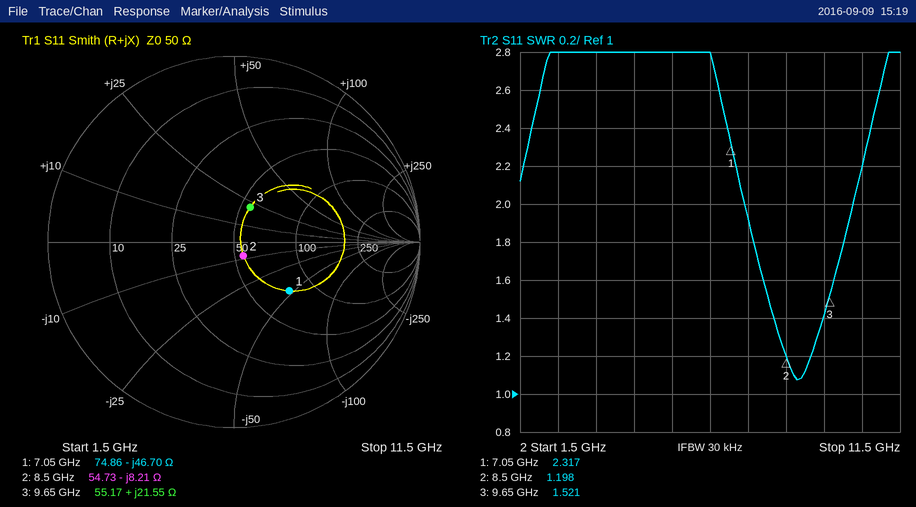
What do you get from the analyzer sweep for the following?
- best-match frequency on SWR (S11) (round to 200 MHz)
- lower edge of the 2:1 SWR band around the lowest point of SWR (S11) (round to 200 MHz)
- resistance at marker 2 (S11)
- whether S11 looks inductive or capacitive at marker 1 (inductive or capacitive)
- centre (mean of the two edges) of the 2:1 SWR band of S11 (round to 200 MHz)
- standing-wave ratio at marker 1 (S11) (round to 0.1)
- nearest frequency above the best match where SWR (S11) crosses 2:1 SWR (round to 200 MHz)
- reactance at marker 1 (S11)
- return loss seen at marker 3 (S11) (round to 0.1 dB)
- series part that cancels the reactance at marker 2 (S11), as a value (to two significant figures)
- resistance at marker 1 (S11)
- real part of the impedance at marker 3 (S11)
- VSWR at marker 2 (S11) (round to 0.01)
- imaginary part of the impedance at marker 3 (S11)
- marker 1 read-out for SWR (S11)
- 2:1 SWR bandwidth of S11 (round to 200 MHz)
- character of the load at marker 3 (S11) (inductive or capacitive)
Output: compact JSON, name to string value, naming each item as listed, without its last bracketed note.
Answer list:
{"best-match frequency on SWR (S11)": "8.8 GHz", "lower edge of the 2:1 SWR band around the lowest point of SWR (S11)": "7.4 GHz", "resistance at marker 2": "54.73 Ω", "whether S11 looks inductive or capacitive at marker 1": "capacitive", "centre (mean of the two edges) of the 2:1 SWR band of S11": "8.8 GHz", "standing-wave ratio at marker 1 (S11)": "2.3", "nearest frequency above the best match where SWR (S11) crosses 2:1 SWR": "10.2 GHz", "reactance at marker 1": "-46.70 Ω", "return loss seen at marker 3 (S11)": "13.7 dB", "series part that cancels the reactance at marker 2 (S11), as a value": "150 pH", "resistance at marker 1": "74.86 Ω", "real part of the impedance at marker 3": "55.17 Ω", "VSWR at marker 2 (S11)": "1.20", "imaginary part of the impedance at marker 3": "+21.55 Ω", "marker 1 read-out for SWR": "2.317", "2:1 SWR bandwidth of S11": "2.8 GHz", "character of the load at marker 3 (S11)": "inductive"}
